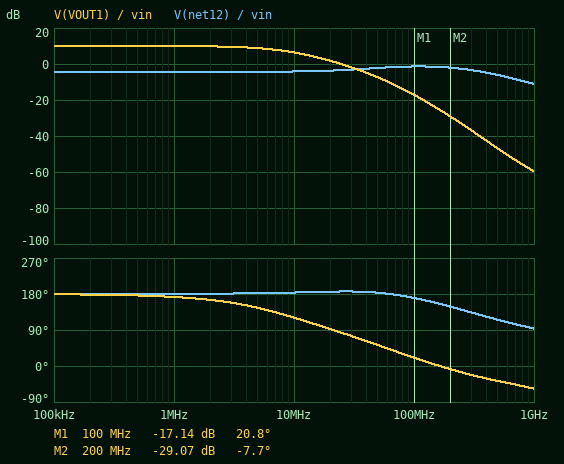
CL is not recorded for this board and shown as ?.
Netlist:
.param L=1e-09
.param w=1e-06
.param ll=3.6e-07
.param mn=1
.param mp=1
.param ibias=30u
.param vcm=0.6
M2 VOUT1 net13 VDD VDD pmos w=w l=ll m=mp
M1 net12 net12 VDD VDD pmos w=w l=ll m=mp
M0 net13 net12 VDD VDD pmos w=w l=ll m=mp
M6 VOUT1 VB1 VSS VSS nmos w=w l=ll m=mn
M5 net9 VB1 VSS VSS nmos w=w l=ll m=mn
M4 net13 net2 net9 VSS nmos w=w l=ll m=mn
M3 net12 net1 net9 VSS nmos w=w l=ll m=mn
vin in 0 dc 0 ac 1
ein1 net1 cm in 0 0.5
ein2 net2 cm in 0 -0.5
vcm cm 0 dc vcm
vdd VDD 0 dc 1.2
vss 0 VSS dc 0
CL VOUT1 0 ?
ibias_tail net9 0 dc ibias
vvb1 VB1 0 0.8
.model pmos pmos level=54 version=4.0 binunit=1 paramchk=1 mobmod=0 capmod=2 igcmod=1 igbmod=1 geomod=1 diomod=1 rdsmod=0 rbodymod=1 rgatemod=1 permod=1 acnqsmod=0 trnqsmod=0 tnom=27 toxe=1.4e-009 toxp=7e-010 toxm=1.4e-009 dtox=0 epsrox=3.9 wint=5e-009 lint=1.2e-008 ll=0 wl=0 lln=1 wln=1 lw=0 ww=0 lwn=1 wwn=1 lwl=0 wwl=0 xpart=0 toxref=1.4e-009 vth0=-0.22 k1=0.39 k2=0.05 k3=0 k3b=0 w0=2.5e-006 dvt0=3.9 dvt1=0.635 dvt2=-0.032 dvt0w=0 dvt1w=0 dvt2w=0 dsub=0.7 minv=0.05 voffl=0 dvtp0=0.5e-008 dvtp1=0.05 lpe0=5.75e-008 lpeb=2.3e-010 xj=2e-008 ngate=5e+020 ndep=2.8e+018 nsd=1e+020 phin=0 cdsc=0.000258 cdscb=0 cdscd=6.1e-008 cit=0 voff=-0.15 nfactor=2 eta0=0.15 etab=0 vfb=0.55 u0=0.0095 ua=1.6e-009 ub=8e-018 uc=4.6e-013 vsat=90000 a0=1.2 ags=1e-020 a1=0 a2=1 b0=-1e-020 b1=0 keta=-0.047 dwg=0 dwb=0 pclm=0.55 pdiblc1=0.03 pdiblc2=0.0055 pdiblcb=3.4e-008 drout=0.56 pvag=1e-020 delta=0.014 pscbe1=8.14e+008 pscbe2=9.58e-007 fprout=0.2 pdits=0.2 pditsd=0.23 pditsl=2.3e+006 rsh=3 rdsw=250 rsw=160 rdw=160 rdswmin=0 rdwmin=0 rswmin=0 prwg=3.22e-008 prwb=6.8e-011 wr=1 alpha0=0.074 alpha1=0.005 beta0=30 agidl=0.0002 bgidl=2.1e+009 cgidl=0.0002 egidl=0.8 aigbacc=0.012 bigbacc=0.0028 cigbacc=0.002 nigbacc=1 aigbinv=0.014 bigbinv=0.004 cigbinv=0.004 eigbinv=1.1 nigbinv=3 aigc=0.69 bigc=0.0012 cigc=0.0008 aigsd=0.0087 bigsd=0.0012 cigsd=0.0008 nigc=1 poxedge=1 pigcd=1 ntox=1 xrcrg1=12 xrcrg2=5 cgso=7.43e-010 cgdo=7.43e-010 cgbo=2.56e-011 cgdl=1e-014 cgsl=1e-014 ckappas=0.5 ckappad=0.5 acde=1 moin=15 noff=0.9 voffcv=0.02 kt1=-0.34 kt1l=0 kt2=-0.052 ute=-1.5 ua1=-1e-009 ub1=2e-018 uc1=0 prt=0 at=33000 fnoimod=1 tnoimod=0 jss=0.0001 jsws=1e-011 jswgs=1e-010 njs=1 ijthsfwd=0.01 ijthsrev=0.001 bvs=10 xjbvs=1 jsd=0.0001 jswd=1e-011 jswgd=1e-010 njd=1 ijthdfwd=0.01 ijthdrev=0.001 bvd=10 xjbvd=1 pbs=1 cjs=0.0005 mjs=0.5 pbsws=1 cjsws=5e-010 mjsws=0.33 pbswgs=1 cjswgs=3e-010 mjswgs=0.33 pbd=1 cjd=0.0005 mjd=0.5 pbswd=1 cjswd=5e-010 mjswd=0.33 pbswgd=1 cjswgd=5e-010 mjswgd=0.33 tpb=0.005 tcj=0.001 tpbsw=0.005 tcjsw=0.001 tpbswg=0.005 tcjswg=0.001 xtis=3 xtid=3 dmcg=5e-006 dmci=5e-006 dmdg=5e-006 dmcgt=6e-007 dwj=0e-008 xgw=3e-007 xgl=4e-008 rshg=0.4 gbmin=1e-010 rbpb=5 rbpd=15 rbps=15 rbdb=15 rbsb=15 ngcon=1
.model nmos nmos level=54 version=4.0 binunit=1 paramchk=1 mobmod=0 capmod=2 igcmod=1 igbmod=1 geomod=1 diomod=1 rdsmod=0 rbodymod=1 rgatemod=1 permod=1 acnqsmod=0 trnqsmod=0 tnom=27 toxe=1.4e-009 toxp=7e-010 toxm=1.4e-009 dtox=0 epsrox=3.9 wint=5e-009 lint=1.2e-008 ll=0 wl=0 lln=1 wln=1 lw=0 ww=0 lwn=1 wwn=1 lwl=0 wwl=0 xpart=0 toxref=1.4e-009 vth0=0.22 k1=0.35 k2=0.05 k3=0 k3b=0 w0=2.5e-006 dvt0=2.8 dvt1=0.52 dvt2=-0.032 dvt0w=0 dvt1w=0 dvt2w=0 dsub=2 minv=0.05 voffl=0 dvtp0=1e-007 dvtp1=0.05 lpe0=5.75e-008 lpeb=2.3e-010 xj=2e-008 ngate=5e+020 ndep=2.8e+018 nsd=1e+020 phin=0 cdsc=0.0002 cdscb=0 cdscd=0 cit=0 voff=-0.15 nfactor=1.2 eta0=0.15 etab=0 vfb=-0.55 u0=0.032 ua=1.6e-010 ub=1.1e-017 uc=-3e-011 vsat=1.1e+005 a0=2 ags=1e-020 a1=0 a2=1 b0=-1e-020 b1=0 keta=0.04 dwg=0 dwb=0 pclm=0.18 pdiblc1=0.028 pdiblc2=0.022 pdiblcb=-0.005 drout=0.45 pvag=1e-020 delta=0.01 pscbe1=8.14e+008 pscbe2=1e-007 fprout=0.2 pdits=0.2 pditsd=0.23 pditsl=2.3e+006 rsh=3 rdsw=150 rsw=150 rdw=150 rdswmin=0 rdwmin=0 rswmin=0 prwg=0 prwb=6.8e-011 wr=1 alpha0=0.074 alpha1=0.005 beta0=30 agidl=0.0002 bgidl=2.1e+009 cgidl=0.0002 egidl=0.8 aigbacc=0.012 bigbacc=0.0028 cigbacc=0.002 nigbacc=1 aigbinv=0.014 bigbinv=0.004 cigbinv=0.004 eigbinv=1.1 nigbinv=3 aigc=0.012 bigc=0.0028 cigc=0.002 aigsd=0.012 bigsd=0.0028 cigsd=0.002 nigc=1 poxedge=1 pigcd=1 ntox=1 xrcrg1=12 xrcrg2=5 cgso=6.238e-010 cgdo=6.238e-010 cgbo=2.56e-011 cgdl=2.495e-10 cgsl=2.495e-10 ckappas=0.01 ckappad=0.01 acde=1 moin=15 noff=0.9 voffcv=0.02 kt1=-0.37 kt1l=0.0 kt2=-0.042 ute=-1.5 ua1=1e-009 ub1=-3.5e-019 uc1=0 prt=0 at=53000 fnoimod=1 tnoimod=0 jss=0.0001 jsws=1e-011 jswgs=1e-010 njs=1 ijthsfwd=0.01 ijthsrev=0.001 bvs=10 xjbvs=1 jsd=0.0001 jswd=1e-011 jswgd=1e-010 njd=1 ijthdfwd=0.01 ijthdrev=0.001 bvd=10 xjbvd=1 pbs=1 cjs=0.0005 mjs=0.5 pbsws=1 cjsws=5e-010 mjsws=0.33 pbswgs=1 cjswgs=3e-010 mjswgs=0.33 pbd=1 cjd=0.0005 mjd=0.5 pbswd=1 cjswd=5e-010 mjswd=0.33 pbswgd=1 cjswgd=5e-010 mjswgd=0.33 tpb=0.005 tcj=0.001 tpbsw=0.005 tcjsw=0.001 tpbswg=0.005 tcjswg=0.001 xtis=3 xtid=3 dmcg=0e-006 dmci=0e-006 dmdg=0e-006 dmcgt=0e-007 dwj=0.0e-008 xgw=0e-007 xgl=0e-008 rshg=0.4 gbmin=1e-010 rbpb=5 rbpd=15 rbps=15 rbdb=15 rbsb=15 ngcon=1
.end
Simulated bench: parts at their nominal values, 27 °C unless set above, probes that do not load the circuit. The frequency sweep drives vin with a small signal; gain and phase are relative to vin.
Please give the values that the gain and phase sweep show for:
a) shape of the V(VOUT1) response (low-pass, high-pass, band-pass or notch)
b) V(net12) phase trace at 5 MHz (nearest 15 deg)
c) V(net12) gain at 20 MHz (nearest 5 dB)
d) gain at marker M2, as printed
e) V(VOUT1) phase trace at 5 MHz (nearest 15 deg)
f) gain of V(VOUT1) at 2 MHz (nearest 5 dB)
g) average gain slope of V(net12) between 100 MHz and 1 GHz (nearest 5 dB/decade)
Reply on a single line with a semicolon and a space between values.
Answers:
low-pass; 180 deg; -5 dB; -29.07 dB; 150 deg; 10 dB; -10 dB/decade
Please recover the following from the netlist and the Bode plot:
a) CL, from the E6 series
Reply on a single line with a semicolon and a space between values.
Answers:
3.3 pF
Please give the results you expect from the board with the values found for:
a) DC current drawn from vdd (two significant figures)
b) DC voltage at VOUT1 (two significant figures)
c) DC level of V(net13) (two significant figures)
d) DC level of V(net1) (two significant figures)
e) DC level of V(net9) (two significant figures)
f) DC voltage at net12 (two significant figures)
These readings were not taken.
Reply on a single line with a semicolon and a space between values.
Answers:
64 µA; 100 mV; 410 mV; 600 mV; 58 mV; 410 mV
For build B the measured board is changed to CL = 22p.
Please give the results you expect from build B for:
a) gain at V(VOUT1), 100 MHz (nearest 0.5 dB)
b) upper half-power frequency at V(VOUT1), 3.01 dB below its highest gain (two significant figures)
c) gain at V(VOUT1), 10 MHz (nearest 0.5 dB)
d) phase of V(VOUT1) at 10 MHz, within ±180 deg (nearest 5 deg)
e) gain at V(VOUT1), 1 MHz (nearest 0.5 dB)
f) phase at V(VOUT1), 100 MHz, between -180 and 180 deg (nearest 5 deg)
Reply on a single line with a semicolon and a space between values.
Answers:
-33.5 dB; 1.4 MHz; -7.5 dB; 85 deg; 8.0 dB; 15 deg
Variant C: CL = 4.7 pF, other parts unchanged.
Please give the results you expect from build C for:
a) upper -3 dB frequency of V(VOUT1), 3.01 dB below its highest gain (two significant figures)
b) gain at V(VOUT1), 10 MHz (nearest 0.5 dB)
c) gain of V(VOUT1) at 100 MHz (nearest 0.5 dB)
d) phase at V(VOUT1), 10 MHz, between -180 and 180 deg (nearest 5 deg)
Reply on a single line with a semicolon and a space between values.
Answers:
6.3 MHz; 4.5 dB; -20.0 dB; 110 deg
